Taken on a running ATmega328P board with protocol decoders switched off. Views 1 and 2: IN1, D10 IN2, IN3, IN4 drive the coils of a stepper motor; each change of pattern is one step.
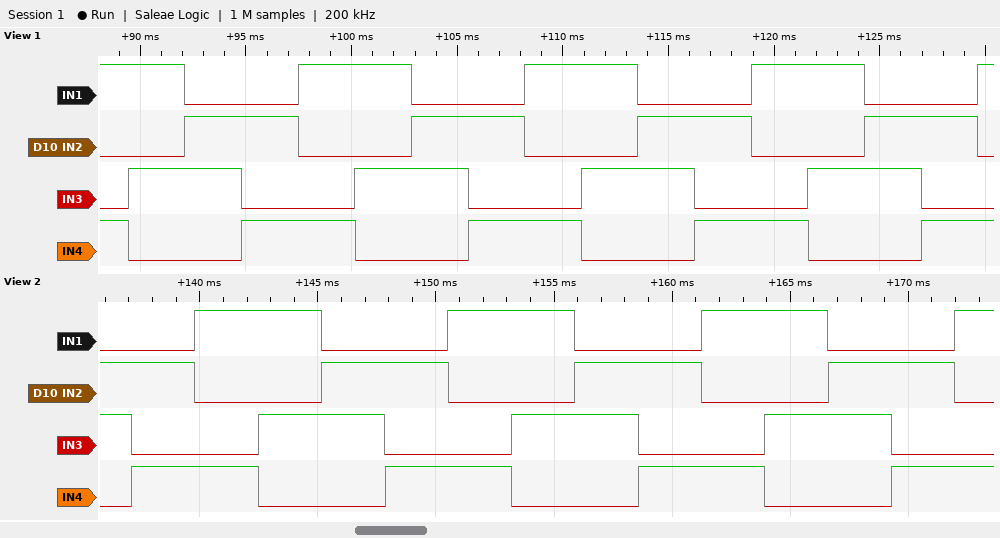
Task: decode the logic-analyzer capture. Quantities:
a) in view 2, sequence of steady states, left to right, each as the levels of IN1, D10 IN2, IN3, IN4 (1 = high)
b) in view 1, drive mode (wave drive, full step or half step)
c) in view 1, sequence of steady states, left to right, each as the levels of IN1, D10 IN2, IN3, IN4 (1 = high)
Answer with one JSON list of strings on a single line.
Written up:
["0110 0101 1001 1010 0110 0101 1001 1010 0110 0101 1001 1010 0110 0101 1001", "full step", "1001 1010 0110 0101 1001 1010 0110 0101 1001 1010 0110 0101 1001 1010 0110 0101 1001"]
